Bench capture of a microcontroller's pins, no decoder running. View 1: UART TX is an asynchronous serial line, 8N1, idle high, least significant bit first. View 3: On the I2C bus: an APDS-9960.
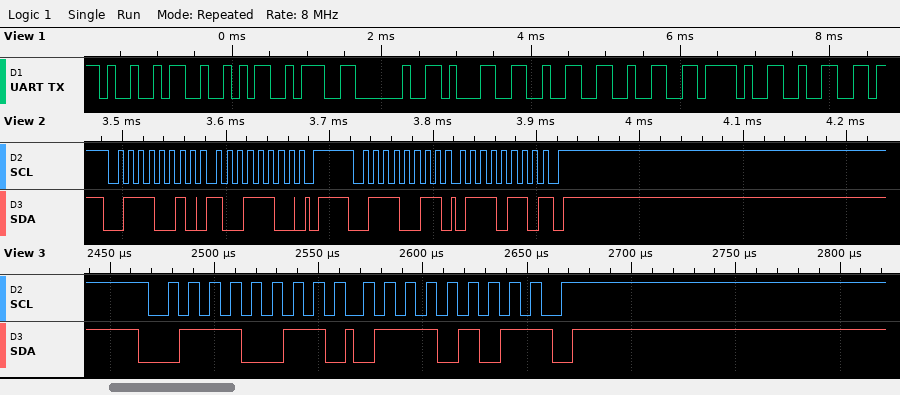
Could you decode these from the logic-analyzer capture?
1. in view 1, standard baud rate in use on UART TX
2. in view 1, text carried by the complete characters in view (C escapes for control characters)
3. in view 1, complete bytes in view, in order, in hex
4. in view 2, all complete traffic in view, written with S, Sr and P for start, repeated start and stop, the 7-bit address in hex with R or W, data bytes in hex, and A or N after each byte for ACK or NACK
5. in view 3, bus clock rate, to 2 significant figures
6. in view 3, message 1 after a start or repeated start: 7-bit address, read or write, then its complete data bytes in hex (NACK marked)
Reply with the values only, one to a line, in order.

9600 baud
"IR: 122/2"
49 52 3A 20 31 32 32 2F 32
S 39W A 9C A P S 39R A 76 N P
100 kHz
0x39 read: 75 NACK
